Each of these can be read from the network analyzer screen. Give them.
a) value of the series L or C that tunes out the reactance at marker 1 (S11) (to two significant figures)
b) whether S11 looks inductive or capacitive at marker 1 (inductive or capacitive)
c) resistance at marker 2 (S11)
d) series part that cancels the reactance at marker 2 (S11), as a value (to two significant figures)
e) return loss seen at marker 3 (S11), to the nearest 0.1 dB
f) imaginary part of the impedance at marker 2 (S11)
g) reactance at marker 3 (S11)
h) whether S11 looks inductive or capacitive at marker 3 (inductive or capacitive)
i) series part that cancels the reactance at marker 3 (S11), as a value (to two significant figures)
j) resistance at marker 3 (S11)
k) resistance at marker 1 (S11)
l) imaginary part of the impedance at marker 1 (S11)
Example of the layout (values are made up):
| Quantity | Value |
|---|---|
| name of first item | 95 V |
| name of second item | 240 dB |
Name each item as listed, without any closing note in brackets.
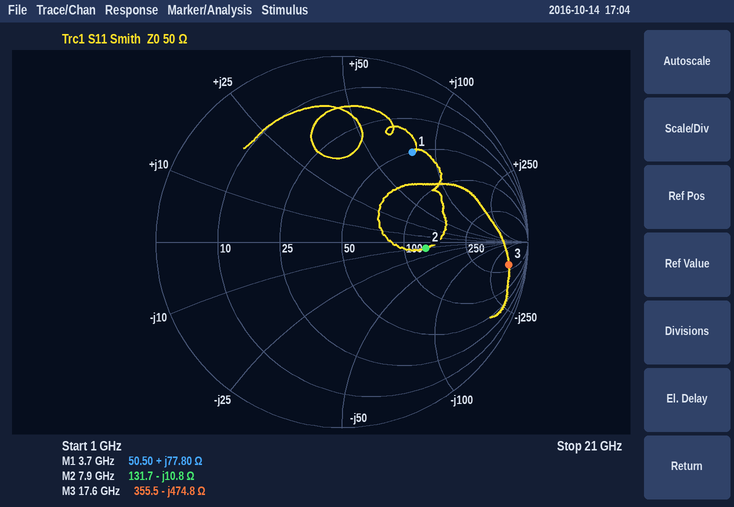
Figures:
| Quantity | Value |
|---|---|
| value of the series L or C that tunes out the reactance at marker 1 (S11) | 550 fF |
| whether S11 looks inductive or capacitive at marker 1 | inductive |
| resistance at marker 2 | 131.7 Ω |
| series part that cancels the reactance at marker 2 (S11), as a value | 220 pH |
| return loss seen at marker 3 (S11), to the nearest 0.1 dB | 0.9 dB |
| imaginary part of the impedance at marker 2 | -10.8 Ω |
| reactance at marker 3 | -474.8 Ω |
| whether S11 looks inductive or capacitive at marker 3 | capacitive |
| series part that cancels the reactance at marker 3 (S11), as a value | 4.3 nH |
| resistance at marker 3 | 355.5 Ω |
| resistance at marker 1 | 50.50 Ω |
| imaginary part of the impedance at marker 1 | +77.80 Ω |
